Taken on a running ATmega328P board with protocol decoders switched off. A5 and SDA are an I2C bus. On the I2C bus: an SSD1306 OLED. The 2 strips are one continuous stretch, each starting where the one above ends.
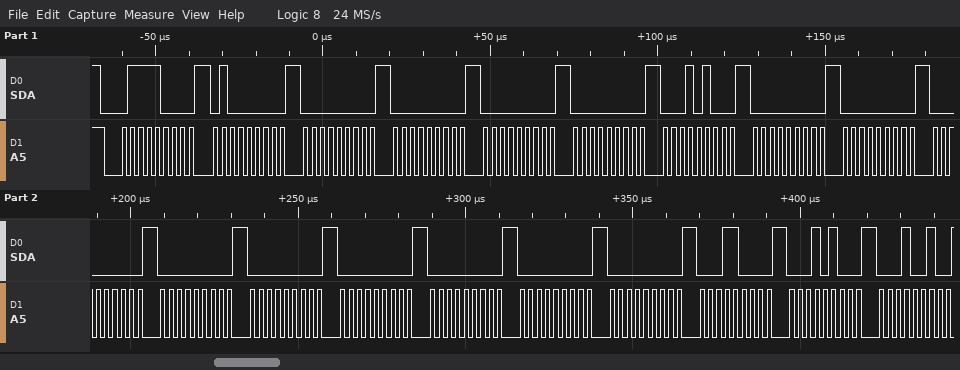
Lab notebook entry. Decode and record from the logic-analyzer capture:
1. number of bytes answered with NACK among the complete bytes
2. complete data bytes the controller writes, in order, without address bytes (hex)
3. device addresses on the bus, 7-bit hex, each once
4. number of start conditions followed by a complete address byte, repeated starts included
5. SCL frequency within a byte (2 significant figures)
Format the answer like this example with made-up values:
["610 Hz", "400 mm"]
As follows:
["0", "40 00 00 00 00 14 00 00 00 00 00 00 00 00 00 18 14 12", "0x3C", "1", "400 kHz"]
